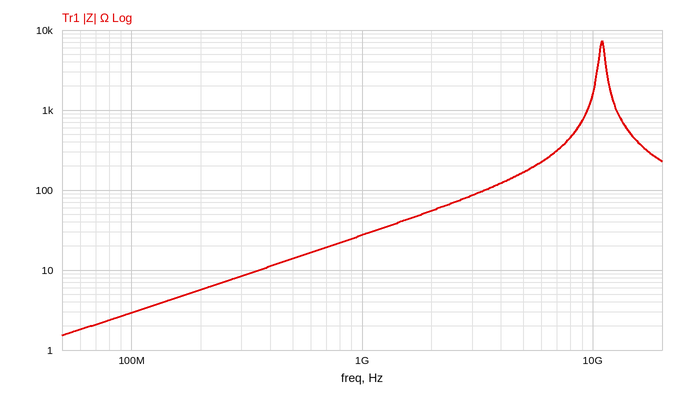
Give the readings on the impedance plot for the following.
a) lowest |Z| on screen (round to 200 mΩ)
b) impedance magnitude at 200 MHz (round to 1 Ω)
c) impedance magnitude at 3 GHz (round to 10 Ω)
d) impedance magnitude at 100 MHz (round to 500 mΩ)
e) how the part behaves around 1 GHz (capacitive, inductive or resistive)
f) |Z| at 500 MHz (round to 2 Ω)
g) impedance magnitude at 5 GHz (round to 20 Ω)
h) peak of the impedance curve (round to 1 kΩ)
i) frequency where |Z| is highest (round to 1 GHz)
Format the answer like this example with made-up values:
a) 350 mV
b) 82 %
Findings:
a) 1.6 Ω
b) 6 Ω
c) 90 Ω
d) 3.0 Ω
e) inductive
f) 14 Ω
g) 160 Ω
h) 7 kΩ
i) 11 GHz
